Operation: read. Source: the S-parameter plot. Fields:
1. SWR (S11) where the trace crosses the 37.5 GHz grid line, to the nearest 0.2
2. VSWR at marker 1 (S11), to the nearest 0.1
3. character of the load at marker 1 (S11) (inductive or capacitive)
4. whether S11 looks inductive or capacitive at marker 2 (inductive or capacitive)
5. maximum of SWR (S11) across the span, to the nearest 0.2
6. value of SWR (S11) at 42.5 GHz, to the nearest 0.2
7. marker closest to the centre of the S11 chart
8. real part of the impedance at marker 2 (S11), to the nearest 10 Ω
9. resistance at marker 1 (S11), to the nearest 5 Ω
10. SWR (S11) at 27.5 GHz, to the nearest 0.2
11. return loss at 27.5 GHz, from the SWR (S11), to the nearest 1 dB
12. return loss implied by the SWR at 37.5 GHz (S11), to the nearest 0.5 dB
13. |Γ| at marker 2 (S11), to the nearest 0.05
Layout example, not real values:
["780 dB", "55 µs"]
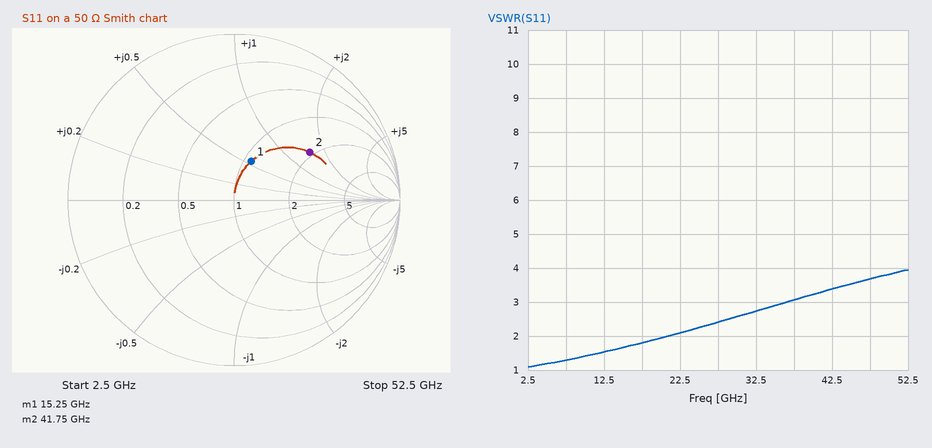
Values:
["3.0", "1.7", "inductive", "inductive", "4.0", "3.4", "marker 1", "90 Ω", "55 Ω", "2.4", "8 dB", "6.0 dB", "0.55"]
